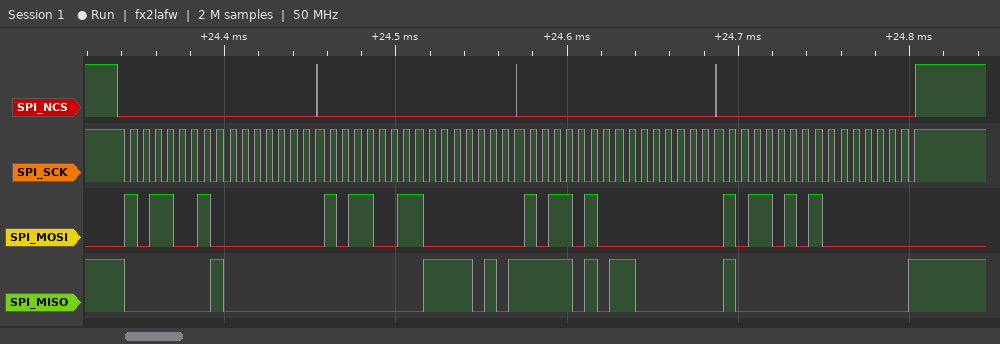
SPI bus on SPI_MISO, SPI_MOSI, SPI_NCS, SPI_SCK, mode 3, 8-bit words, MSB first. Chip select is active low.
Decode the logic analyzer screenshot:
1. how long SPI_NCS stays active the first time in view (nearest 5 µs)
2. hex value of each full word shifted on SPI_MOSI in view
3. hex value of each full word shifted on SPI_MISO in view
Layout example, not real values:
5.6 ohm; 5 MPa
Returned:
115 µs; B2, 00, B3, 00, B4, 00, B5, 00; 01, 00, 00, F5, F5, 80, 80, 01
